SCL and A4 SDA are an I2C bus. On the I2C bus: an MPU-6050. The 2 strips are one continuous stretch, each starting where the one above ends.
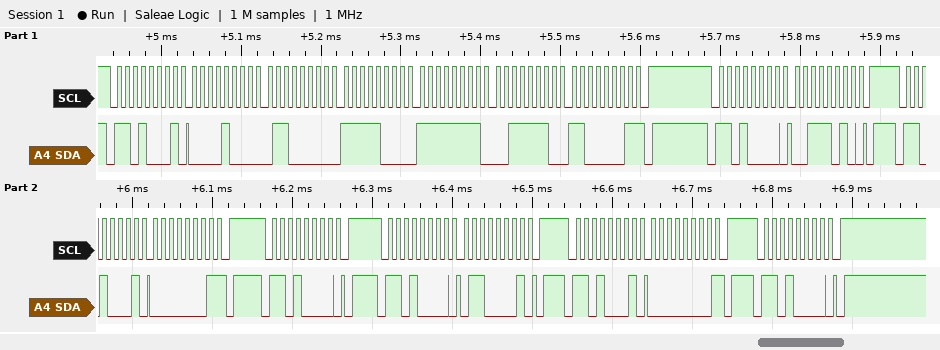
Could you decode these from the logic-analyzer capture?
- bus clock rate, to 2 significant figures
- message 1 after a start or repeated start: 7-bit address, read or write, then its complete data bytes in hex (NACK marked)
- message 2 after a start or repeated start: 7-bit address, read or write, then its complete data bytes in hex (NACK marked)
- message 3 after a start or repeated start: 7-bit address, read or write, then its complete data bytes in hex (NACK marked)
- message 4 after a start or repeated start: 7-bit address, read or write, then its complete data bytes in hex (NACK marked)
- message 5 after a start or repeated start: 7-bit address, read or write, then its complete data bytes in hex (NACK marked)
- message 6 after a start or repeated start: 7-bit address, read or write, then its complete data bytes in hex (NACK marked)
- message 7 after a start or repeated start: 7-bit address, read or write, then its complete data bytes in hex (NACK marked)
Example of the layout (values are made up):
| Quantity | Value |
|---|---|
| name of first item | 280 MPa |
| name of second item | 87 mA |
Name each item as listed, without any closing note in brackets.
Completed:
| Quantity | Value |
|---|---|
| bus clock rate, to 2 significant figures | 100 kHz |
| message 1 after a start or repeated start: 7-bit address, read or write, then its complete data bytes in hex | 0x68 read: 08 60 F8 FF 3E C1 NACK |
| message 2 after a start or repeated start: 7-bit address, read or write, then its complete data bytes in hex | 0x68 write: 3A |
| message 3 after a start or repeated start: 7-bit address, read or write, then its complete data bytes in hex | 0x68 read: 01 NACK |
| message 4 after a start or repeated start: 7-bit address, read or write, then its complete data bytes in hex | 0x68 write |
| message 5 after a start or repeated start: 7-bit address, read or write, then its complete data bytes in hex | 0x68 write: 61 |
| message 6 after a start or repeated start: 7-bit address, read or write, then its complete data bytes in hex | 0x68 read: 00 NACK |
| message 7 after a start or repeated start: 7-bit address, read or write, then its complete data bytes in hex | 0x68 write |
